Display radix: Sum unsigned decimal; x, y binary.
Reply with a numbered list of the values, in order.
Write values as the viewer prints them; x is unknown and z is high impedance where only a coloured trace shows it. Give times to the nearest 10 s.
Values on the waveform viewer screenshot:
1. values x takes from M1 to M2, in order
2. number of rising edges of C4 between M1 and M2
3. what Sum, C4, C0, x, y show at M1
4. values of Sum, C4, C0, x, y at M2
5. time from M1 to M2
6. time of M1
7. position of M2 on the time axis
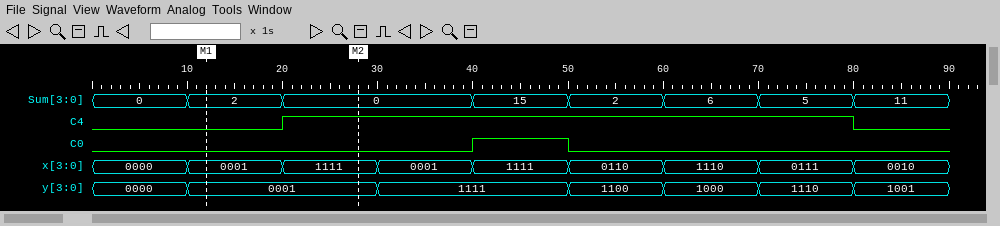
1. 0001, 1111
2. 1
3. Sum=2, C4=0, C0=0, x=0001, y=0001
4. Sum=0, C4=1, C0=0, x=1111, y=0001
5. 20 s
6. 10 s
7. 30 s
